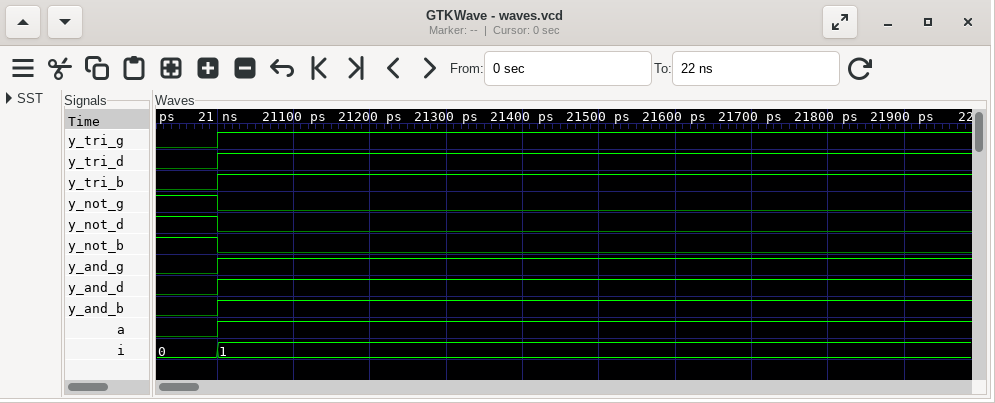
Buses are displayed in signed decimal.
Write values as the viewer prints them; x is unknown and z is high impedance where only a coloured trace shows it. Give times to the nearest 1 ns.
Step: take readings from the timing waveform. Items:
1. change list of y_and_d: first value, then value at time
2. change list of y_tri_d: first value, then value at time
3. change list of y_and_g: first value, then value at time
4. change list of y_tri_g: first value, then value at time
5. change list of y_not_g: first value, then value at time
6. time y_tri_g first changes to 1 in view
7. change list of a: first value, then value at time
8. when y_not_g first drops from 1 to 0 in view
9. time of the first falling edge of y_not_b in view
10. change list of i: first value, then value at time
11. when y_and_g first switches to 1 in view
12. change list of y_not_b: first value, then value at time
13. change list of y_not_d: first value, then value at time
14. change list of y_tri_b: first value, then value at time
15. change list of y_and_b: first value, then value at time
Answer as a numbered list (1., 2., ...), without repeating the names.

1. 0, 1 at 21 ns
2. 0, 1 at 21 ns
3. 0, 1 at 21 ns
4. 0, 1 at 21 ns
5. 1, 0 at 21 ns
6. 21 ns
7. 0, 1 at 21 ns
8. 21 ns
9. 21 ns
10. 0, 1 at 21 ns
11. 21 ns
12. 1, 0 at 21 ns
13. 1, 0 at 21 ns
14. 0, 1 at 21 ns
15. 0, 1 at 21 ns
